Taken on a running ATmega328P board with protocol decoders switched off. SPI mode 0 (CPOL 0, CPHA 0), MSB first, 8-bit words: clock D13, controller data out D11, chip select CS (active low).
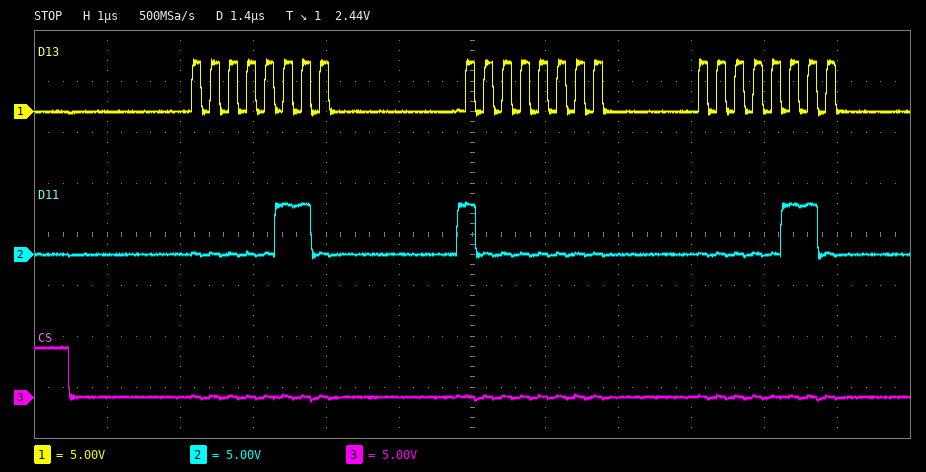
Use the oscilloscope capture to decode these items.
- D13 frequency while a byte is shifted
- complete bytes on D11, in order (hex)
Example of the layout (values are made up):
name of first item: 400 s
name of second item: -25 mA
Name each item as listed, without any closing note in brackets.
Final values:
D13 frequency while a byte is shifted: 4 MHz
complete bytes on D11, in order: 06 80 06
